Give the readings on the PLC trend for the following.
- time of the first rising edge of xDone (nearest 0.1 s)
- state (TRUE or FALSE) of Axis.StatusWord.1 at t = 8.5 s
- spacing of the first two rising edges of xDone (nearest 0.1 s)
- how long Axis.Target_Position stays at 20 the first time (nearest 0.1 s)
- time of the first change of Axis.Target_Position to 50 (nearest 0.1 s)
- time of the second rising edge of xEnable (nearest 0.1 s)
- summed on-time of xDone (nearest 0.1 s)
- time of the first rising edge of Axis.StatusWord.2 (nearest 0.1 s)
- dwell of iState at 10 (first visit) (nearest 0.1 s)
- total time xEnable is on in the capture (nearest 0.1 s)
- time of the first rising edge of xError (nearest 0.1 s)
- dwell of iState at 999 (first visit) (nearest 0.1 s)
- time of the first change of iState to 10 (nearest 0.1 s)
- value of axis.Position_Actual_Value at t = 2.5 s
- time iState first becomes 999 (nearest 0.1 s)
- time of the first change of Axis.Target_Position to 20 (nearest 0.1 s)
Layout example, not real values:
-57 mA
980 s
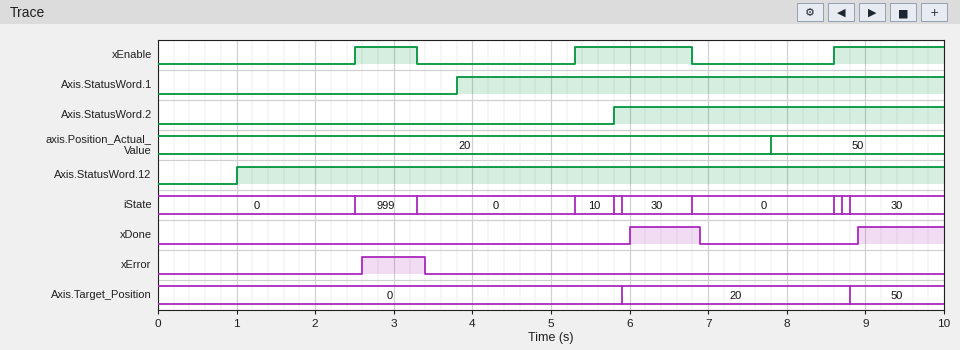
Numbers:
6.0 s
TRUE
2.9 s
2.9 s
8.8 s
5.3 s
2.0 s
5.8 s
0.5 s
3.7 s
2.6 s
0.8 s
5.3 s
20
2.5 s
5.9 s
